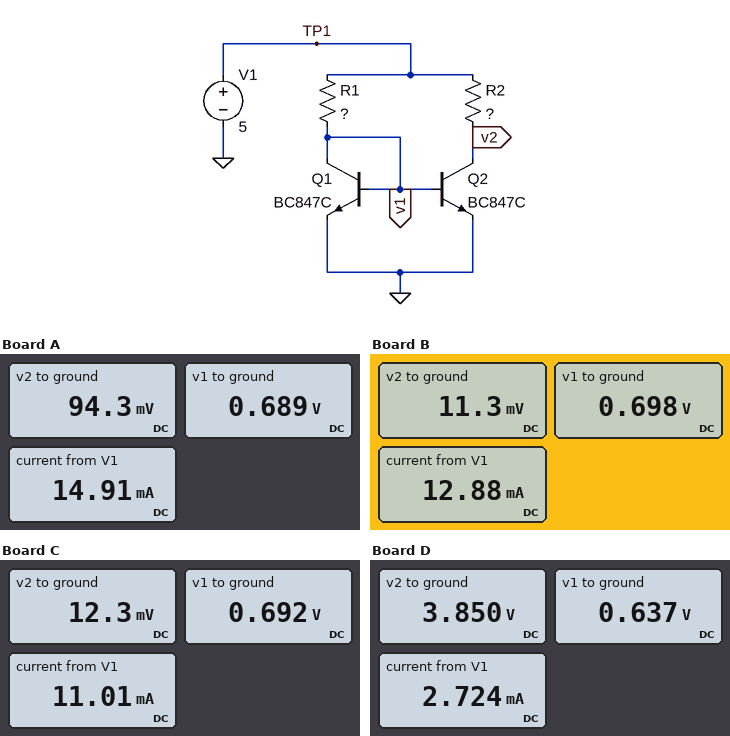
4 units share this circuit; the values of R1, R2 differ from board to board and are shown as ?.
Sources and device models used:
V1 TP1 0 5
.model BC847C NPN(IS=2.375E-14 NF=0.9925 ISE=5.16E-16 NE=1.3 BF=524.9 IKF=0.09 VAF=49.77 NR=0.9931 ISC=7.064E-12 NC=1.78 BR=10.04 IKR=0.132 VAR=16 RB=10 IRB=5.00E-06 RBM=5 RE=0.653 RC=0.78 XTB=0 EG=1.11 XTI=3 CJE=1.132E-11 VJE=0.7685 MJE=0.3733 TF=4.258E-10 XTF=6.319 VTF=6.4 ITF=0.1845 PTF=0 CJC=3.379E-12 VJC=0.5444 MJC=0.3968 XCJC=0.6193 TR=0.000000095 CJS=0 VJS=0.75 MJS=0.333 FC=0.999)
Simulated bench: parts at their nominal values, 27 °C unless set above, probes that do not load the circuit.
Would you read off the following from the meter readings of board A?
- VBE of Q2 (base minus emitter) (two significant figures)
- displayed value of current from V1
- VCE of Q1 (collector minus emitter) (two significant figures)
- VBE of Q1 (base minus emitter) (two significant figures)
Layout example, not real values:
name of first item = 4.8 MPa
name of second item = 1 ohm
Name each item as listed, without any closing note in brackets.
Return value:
VBE of Q2 (base minus emitter) = 690 mV
displayed value of current from V1 = 14.91 mA
VCE of Q1 (collector minus emitter) = 690 mV
VBE of Q1 (base minus emitter) = 690 mV
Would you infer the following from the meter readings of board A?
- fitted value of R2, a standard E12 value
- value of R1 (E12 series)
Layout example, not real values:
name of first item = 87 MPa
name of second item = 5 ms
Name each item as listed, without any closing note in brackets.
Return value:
fitted value of R2, a standard E12 value = 680 Ω
value of R1 = 560 Ω
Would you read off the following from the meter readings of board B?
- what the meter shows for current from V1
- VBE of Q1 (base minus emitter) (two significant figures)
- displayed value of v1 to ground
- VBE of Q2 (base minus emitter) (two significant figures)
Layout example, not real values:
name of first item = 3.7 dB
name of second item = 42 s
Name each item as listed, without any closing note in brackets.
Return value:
what the meter shows for current from V1 = 12.88 mA
VBE of Q1 (base minus emitter) = 700 mV
displayed value of v1 to ground = 0.698 V
VBE of Q2 (base minus emitter) = 700 mV
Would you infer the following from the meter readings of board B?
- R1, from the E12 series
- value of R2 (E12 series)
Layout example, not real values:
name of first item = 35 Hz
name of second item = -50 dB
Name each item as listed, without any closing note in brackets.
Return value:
R1, from the E12 series = 390 Ω
value of R2 = 2.7 kΩ
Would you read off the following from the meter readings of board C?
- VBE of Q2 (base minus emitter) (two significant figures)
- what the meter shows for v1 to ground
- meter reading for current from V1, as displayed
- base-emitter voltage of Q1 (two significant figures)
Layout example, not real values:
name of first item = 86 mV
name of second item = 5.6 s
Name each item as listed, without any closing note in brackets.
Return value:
VBE of Q2 (base minus emitter) = 690 mV
what the meter shows for v1 to ground = 0.692 V
meter reading for current from V1, as displayed = 11.01 mA
base-emitter voltage of Q1 = 690 mV
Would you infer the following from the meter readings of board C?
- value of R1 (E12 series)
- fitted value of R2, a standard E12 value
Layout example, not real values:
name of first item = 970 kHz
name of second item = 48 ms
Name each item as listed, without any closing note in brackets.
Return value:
value of R1 = 470 Ω
fitted value of R2, a standard E12 value = 2.7 kΩ
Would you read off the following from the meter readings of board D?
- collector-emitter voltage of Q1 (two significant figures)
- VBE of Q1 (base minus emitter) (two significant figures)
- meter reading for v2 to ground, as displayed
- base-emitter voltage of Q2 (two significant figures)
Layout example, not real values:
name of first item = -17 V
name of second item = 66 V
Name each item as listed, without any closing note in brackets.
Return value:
collector-emitter voltage of Q1 = 640 mV
VBE of Q1 (base minus emitter) = 640 mV
meter reading for v2 to ground, as displayed = 3.850 V
base-emitter voltage of Q2 = 640 mV
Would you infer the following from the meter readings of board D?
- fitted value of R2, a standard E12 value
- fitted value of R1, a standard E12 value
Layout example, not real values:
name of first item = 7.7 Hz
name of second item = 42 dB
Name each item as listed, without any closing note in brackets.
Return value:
fitted value of R2, a standard E12 value = 820 Ω
fitted value of R1, a standard E12 value = 3.3 kΩ
